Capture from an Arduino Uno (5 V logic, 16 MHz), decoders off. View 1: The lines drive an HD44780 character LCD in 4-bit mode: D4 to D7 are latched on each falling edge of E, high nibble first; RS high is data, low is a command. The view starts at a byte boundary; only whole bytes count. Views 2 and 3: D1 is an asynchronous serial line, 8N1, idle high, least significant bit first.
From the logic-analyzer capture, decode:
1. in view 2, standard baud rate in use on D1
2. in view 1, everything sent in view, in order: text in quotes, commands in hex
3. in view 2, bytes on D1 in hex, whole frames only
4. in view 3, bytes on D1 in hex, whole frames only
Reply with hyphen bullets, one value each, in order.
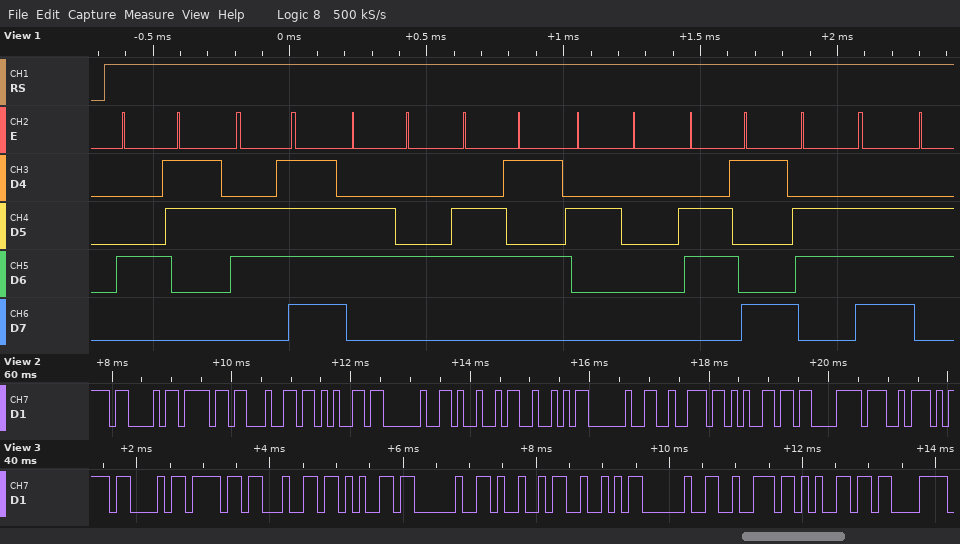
- 9600 baud
- "Code in"
- 43 6F 64 65 20 49 52 20 72 65 C3 A7
- 43 6F 64 65 20 49 52 20 72 65 C3
